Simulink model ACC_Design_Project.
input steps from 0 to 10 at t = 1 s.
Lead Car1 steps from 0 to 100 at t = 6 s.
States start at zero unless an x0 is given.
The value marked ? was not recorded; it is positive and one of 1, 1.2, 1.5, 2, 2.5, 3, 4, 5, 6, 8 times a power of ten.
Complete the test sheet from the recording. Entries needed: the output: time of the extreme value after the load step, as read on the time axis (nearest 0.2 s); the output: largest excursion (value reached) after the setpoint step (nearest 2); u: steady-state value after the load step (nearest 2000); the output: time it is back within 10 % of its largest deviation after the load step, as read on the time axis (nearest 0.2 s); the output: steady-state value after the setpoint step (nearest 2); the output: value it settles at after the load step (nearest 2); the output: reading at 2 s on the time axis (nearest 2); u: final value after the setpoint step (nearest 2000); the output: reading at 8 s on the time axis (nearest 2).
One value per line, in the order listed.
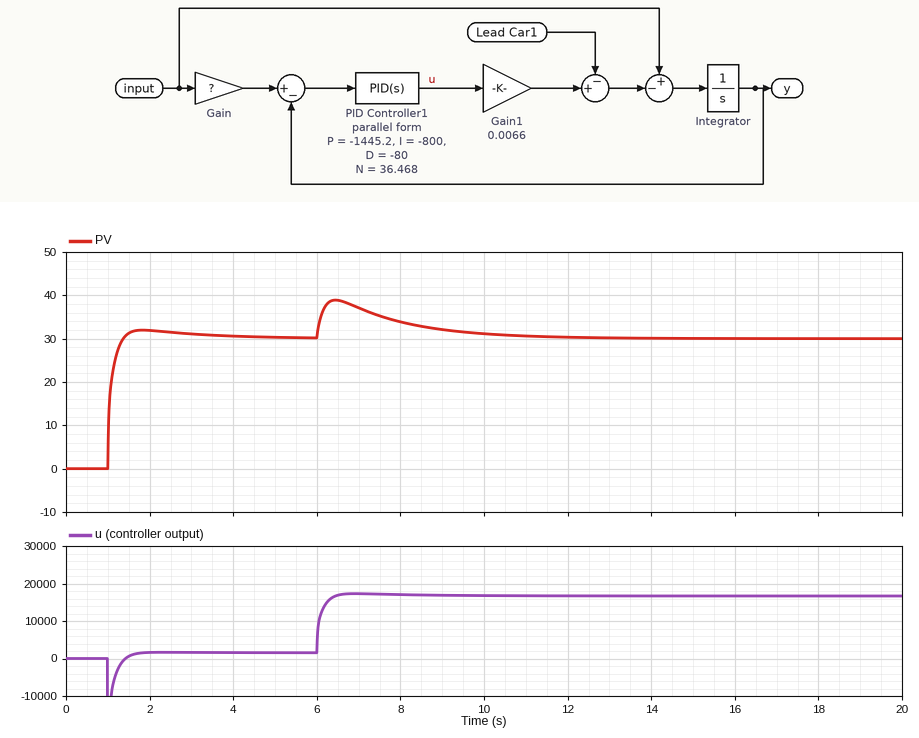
6.4 s
32
16000
10.4 s
30
30
32
2000
34
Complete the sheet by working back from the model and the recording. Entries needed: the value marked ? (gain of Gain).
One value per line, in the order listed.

3
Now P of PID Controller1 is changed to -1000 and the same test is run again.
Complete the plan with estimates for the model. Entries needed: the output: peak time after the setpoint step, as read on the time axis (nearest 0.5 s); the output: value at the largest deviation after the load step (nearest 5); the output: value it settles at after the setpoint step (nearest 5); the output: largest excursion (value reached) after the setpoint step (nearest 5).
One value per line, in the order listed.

2.0 s
40
30
35
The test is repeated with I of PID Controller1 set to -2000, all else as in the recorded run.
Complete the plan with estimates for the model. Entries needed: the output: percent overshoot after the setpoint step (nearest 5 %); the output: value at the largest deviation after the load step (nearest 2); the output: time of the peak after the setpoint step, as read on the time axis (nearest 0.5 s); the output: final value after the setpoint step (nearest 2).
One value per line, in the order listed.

10 %
38
1.5 s
30
